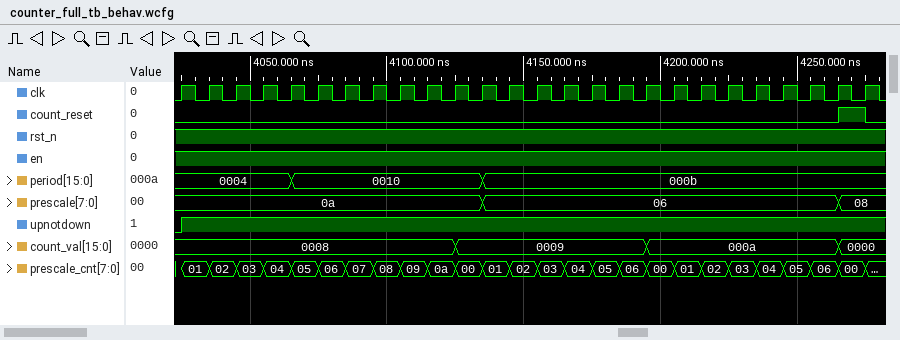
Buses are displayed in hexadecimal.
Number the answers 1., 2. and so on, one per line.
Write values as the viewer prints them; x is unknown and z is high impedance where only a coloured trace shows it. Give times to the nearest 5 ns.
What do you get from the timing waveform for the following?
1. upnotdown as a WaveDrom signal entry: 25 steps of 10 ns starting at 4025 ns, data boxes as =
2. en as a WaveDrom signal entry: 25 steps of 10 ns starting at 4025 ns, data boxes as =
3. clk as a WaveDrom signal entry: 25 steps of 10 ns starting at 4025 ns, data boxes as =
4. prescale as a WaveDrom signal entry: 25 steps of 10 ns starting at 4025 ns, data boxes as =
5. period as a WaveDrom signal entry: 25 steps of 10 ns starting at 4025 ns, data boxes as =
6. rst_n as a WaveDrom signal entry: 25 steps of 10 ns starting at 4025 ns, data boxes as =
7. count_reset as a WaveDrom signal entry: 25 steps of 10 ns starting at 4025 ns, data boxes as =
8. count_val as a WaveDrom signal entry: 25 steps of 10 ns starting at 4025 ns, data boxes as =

1. {name: 'upnotdown', wave: '1........................'}
2. {name: 'en', wave: '1........................'}
3. {name: 'clk', wave: 'p........................'}
4. {name: 'prescale', wave: '=..........=............=', data: '0a 06 08'}
5. {name: 'period', wave: '=...=......=.............', data: '0004 0010 000b'}
6. {name: 'rst_n', wave: '1........................'}
7. {name: 'count_reset', wave: '0.......................1'}
8. {name: 'count_val', wave: '=.........=......=......=', data: '0008 0009 000a 0000'}
